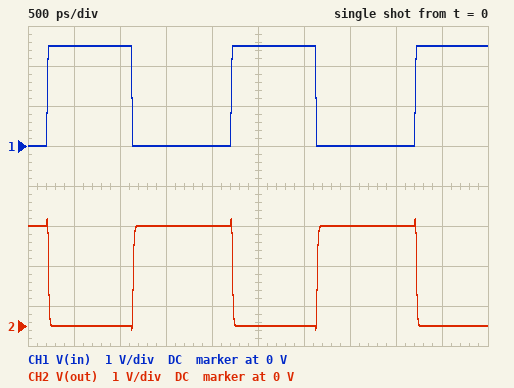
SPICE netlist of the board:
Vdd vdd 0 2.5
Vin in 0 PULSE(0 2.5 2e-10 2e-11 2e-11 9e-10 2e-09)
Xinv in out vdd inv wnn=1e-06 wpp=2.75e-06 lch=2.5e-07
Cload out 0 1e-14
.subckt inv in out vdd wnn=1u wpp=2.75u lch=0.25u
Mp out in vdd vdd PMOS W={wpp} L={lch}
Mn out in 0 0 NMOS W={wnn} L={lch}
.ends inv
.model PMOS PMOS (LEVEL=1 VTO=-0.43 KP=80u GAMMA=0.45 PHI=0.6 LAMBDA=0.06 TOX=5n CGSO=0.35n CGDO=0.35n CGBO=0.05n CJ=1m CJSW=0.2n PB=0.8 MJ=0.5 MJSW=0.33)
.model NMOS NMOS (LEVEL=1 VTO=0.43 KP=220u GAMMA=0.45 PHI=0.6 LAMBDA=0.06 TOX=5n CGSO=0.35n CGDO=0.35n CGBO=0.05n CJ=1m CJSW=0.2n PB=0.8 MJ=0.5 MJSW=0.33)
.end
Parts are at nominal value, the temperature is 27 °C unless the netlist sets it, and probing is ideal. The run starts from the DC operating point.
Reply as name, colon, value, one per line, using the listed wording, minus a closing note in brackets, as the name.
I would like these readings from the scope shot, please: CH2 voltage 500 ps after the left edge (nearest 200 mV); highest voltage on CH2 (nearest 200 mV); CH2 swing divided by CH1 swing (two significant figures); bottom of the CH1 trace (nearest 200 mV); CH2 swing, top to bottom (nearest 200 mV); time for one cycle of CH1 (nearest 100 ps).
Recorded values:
CH2 voltage 500 ps after the left edge: 0 V
highest voltage on CH2: 2.6 V
CH2 swing divided by CH1 swing: 1.1
bottom of the CH1 trace: 0 V
CH2 swing, top to bottom: 2.8 V
time for one cycle of CH1: 2.0 ns
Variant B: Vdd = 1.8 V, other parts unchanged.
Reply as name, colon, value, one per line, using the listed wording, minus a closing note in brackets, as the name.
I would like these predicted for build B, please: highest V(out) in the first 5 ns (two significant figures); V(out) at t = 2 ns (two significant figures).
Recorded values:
highest V(out) in the first 5 ns: 2.0 V
V(out) at t = 2 ns: 1.8 V
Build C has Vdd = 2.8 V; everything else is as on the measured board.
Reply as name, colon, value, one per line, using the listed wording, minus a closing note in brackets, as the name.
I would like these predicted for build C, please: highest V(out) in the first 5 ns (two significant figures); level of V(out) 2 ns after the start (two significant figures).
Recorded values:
highest V(out) in the first 5 ns: 3.0 V
level of V(out) 2 ns after the start: 2.8 V
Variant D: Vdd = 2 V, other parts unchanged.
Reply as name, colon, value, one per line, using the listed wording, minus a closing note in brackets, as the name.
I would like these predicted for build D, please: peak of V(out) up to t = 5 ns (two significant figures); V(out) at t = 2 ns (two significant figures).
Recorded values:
peak of V(out) up to t = 5 ns: 2.2 V
V(out) at t = 2 ns: 2.0 V
